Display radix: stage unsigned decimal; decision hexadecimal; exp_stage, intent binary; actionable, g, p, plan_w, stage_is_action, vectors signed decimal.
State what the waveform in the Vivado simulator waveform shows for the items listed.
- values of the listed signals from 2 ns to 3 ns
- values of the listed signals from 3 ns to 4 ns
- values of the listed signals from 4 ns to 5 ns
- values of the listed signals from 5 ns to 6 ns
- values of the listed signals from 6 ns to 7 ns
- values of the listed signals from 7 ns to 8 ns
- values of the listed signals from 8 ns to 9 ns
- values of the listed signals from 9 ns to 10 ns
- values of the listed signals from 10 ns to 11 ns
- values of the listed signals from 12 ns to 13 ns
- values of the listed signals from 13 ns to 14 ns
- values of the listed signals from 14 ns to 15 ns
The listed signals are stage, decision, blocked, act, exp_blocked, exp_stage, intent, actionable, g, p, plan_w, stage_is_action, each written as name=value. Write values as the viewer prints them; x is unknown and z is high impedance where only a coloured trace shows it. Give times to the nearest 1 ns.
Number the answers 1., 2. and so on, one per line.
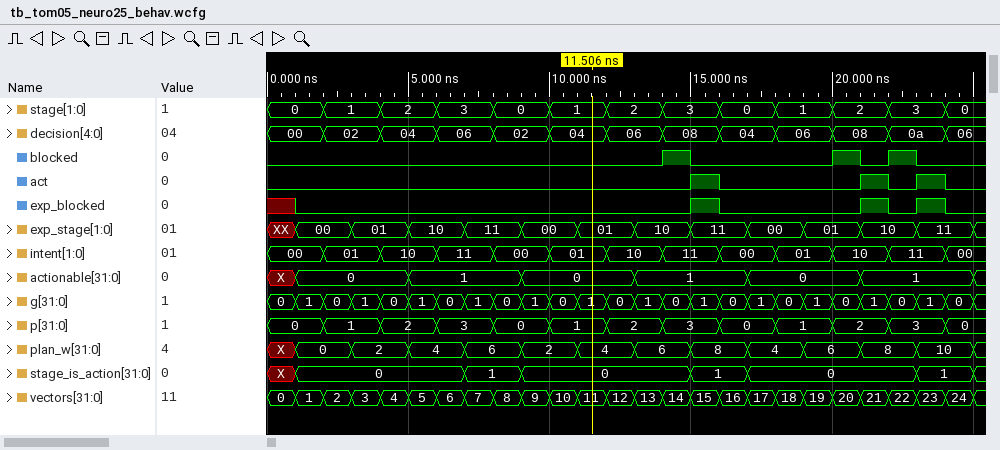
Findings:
1. stage=1, decision=02, blocked=0, act=0, exp_blocked=0, exp_stage=00, intent=01, actionable=0, g=0, p=1, plan_w=0, stage_is_action=0
2. stage=1, decision=02, blocked=0, act=0, exp_blocked=0, exp_stage=01, intent=01, actionable=0, g=1, p=1, plan_w=2, stage_is_action=0
3. stage=2, decision=04, blocked=0, act=0, exp_blocked=0, exp_stage=01, intent=10, actionable=0, g=0, p=2, plan_w=2, stage_is_action=0
4. stage=2, decision=04, blocked=0, act=0, exp_blocked=0, exp_stage=10, intent=10, actionable=1, g=1, p=2, plan_w=4, stage_is_action=0
5. stage=3, decision=06, blocked=0, act=0, exp_blocked=0, exp_stage=10, intent=11, actionable=1, g=0, p=3, plan_w=4, stage_is_action=0
6. stage=3, decision=06, blocked=0, act=0, exp_blocked=0, exp_stage=11, intent=11, actionable=1, g=1, p=3, plan_w=6, stage_is_action=1
7. stage=0, decision=02, blocked=0, act=0, exp_blocked=0, exp_stage=11, intent=00, actionable=1, g=0, p=0, plan_w=6, stage_is_action=1
8. stage=0, decision=02, blocked=0, act=0, exp_blocked=0, exp_stage=00, intent=00, actionable=0, g=1, p=0, plan_w=2, stage_is_action=0
9. stage=1, decision=04, blocked=0, act=0, exp_blocked=0, exp_stage=00, intent=01, actionable=0, g=0, p=1, plan_w=2, stage_is_action=0
10. stage=2, decision=06, blocked=0, act=0, exp_blocked=0, exp_stage=01, intent=10, actionable=0, g=0, p=2, plan_w=4, stage_is_action=0
11. stage=2, decision=06, blocked=0, act=0, exp_blocked=0, exp_stage=10, intent=10, actionable=1, g=1, p=2, plan_w=6, stage_is_action=0
12. stage=3, decision=08, blocked=1, act=0, exp_blocked=0, exp_stage=10, intent=11, actionable=1, g=0, p=3, plan_w=6, stage_is_action=0
